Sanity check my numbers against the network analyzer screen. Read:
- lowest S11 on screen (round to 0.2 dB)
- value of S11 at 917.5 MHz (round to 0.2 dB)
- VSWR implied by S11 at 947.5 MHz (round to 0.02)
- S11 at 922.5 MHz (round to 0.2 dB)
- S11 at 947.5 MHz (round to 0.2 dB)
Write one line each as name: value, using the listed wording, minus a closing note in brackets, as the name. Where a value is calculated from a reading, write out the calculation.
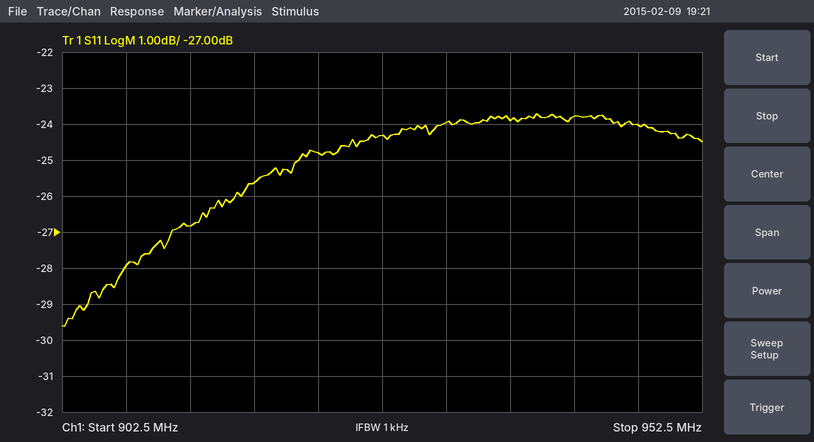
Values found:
lowest S11 on screen: -29.6 dB
value of S11 at 917.5 MHz: -25.6 dB
VSWR implied by S11 at 947.5 MHz: |Γ| = 10^(-24/20) = 0.0631; VSWR = (1 + 0.0631)/(1 − 0.0631) ≈ 1.13, so 1.14 to the nearest 0.02
S11 at 922.5 MHz: -24.8 dB
S11 at 947.5 MHz: -24.0 dB
